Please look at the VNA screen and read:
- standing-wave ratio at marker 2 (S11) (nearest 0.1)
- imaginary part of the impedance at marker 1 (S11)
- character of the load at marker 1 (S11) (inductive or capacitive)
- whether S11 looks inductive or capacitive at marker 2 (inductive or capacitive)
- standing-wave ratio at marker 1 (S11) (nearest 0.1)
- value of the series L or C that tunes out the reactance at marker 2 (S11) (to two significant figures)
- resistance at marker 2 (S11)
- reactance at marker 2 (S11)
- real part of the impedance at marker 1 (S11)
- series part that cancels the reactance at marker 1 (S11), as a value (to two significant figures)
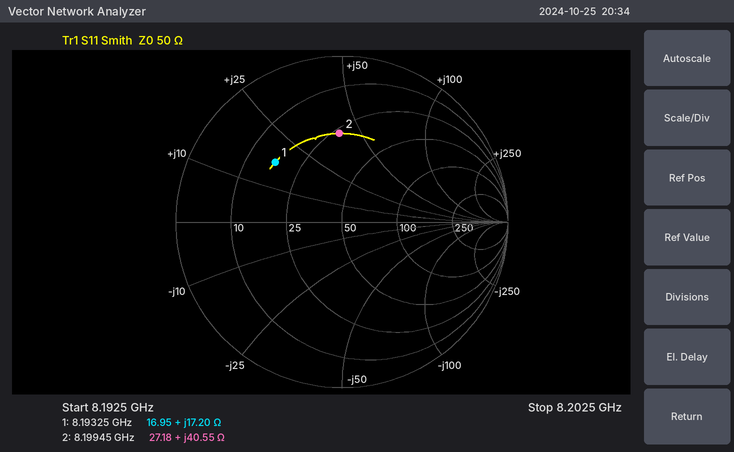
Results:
3.3
+17.20 Ω
inductive
inductive
3.3
480 fF
27.18 Ω
+40.55 Ω
16.95 Ω
1.1 pF
